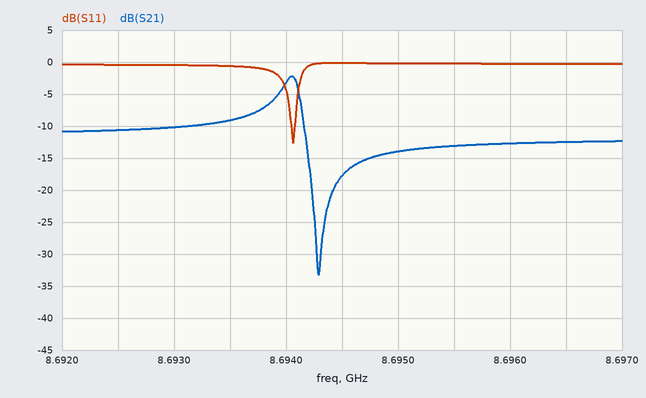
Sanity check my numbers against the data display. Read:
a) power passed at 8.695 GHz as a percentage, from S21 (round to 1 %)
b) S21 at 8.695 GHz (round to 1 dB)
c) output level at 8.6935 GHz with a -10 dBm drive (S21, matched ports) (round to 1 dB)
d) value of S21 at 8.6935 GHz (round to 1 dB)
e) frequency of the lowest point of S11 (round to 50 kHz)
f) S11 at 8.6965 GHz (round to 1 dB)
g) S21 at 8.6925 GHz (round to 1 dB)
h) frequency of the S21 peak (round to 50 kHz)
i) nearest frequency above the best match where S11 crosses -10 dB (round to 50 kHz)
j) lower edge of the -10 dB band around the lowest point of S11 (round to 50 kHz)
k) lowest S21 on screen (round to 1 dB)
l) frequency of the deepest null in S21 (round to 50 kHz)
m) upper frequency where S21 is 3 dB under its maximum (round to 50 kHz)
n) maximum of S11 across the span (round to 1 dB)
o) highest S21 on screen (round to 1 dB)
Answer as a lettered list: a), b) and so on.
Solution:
a) 4 %
b) -14 dB
c) -19 dBm
d) -9 dB
e) 8.69405 GHz
f) 0 dB
g) -11 dB
h) 8.69405 GHz
i) 8.69410 GHz
j) 8.69405 GHz
k) -33 dB
l) 8.69430 GHz
m) 8.69410 GHz
n) 0 dB
o) -2 dB
